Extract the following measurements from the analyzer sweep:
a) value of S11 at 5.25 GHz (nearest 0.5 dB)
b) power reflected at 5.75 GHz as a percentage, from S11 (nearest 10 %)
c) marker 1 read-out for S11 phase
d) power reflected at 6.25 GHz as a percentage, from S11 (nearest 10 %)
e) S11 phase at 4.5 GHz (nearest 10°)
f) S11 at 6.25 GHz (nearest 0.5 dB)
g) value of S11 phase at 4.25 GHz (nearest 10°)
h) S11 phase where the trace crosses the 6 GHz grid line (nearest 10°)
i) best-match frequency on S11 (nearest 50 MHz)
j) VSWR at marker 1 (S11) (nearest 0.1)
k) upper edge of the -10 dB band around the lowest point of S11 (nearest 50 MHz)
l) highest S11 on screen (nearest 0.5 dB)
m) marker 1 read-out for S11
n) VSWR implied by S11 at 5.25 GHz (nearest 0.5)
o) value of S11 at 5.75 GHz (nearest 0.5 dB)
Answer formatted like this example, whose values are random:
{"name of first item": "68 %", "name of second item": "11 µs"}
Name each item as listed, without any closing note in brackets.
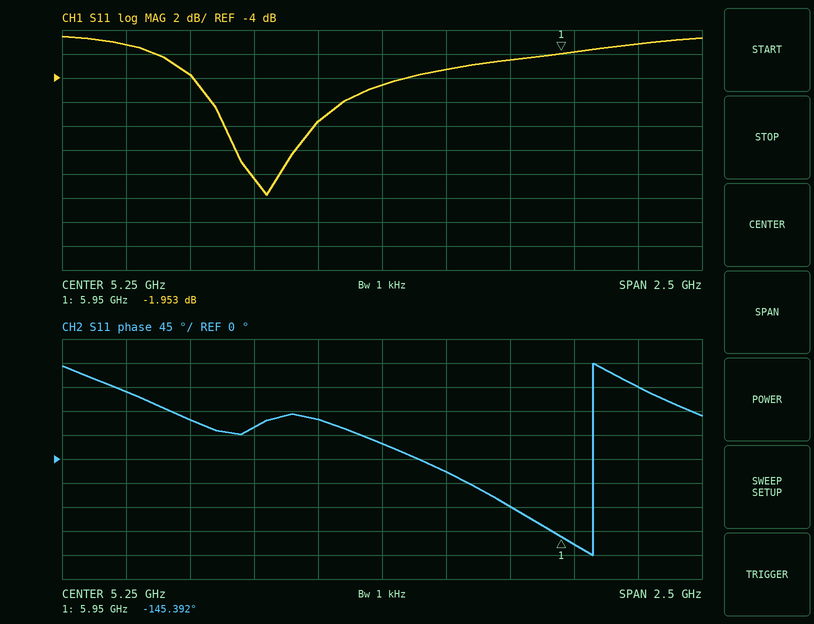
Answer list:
{"value of S11 at 5.25 GHz": "-4.5 dB", "power reflected at 5.75 GHz as a percentage, from S11": "60 %", "marker 1 read-out for S11 phase": "-145.392°", "power reflected at 6.25 GHz as a percentage, from S11": "80 %", "S11 phase at 4.5 GHz": "70°", "S11 at 6.25 GHz": "-1.0 dB", "value of S11 phase at 4.25 GHz": "130°", "S11 phase where the trace crosses the 6 GHz grid line": "-160°", "best-match frequency on S11": "4.80 GHz", "VSWR at marker 1 (S11)": "8.9", "upper edge of the -10 dB band around the lowest point of S11": "4.90 GHz", "highest S11 on screen": "-0.5 dB", "marker 1 read-out for S11": "-1.953 dB", "VSWR implied by S11 at 5.25 GHz": "4.0", "value of S11 at 5.75 GHz": "-2.5 dB"}
